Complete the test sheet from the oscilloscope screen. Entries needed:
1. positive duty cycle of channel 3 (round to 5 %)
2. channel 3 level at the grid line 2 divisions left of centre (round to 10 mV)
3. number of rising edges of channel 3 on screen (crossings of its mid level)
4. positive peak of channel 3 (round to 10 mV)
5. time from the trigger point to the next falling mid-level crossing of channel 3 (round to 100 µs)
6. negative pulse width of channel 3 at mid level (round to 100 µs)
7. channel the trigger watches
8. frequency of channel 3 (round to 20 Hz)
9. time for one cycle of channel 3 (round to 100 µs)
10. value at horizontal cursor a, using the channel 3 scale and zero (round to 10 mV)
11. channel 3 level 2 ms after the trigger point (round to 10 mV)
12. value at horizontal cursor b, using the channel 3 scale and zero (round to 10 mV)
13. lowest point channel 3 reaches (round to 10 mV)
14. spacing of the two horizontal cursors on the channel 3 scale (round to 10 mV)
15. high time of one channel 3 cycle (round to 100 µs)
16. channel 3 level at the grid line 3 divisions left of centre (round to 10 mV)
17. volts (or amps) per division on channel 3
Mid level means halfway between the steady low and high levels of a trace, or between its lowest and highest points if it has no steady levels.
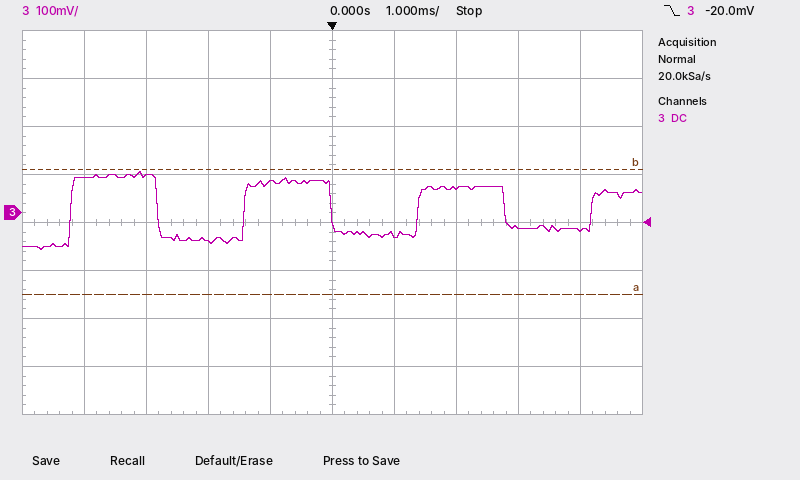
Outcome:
50 %
-60 mV
4
90 mV
2.8 ms
1.4 ms
channel 3
360 Hz
2.8 ms
-170 mV
50 mV
90 mV
-80 mV
260 mV
1.4 ms
80 mV
100 mV
